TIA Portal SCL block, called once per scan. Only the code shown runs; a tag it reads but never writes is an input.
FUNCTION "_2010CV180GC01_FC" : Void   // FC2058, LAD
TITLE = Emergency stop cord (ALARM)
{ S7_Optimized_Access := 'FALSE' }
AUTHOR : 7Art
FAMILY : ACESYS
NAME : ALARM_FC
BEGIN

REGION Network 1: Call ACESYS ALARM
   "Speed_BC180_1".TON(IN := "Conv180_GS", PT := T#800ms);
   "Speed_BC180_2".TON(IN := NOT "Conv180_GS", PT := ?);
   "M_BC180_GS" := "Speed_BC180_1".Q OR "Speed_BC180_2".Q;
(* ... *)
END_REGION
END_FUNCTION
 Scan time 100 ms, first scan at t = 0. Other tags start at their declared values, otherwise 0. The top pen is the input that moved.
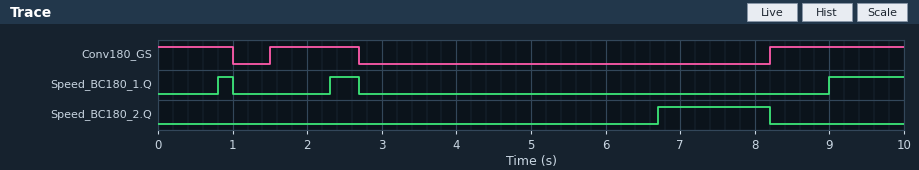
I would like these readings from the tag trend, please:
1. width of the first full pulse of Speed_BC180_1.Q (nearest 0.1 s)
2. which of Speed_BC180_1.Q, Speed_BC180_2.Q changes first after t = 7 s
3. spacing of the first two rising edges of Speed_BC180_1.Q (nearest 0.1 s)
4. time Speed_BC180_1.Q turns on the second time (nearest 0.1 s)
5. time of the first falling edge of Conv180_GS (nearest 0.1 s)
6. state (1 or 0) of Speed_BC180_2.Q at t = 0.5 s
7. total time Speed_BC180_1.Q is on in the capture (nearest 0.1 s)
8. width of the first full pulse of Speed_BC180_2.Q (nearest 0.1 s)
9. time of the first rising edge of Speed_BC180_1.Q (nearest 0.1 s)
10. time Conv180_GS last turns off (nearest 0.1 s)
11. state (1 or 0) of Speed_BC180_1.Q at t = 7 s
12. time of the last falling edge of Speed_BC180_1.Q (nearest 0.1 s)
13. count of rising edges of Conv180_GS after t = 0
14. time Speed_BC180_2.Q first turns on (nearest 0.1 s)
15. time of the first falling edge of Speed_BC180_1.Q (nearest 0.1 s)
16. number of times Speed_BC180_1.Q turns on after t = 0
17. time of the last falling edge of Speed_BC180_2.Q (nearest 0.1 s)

0.2 s
Speed_BC180_2.Q
1.5 s
2.3 s
1.0 s
0
1.6 s
1.5 s
0.8 s
2.7 s
0
2.7 s
2
6.7 s
1.0 s
3
8.2 s
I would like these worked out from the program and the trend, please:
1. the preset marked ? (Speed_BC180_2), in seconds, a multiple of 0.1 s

4.0 s
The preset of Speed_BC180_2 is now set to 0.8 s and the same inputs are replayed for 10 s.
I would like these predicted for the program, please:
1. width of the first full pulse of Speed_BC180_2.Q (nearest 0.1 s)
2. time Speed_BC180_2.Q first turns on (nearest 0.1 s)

4.7 s
3.5 s
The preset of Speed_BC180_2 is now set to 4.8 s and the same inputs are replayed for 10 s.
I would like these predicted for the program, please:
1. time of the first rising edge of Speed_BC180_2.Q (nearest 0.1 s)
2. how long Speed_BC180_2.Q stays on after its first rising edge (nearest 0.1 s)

7.5 s
0.7 s
